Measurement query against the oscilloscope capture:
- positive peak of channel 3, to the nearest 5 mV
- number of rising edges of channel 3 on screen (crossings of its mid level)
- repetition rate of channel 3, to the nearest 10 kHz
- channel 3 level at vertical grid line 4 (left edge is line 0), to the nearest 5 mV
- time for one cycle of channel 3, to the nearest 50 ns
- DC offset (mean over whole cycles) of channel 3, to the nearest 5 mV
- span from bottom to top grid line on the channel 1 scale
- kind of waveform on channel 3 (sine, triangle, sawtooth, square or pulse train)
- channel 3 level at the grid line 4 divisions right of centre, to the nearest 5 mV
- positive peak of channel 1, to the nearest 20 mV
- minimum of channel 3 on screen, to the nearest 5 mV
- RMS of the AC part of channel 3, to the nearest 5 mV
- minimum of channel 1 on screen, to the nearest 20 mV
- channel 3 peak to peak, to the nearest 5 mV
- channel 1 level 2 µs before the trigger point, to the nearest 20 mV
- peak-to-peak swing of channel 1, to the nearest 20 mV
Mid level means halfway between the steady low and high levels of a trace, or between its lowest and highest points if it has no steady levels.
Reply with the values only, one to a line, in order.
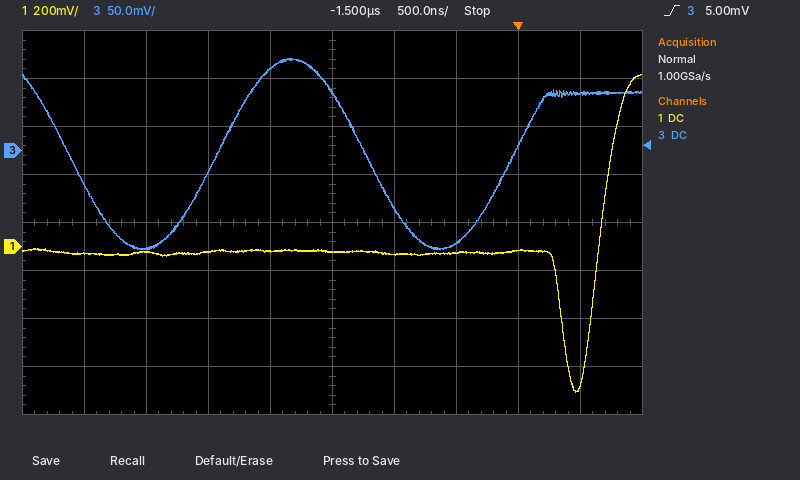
95 mV
2
420 kHz
85 mV
2.40 µs
-5 mV
1.6 V
sine
60 mV
720 mV
-105 mV
70 mV
-600 mV
200 mV
-20 mV
1.32 V
